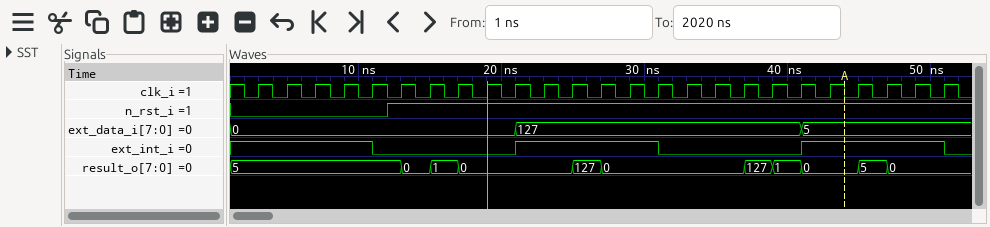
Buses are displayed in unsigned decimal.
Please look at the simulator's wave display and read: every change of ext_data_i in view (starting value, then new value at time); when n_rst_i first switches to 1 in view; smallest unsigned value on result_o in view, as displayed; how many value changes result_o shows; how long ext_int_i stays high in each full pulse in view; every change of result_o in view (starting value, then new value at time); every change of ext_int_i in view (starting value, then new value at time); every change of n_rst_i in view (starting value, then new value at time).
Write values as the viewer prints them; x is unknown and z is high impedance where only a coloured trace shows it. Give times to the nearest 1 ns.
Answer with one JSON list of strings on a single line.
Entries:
["0, 127 at 21 ns, 5 at 41 ns", "12 ns", "0", "10", "10 ns, 10 ns", "5, 0 at 13 ns, 1 at 15 ns, 0 at 17 ns, 127 at 25 ns, 0 at 27 ns, 127 at 37 ns, 1 at 39 ns, 0 at 41 ns, 5 at 45 ns, 0 at 47 ns", "1, 0 at 11 ns, 1 at 21 ns, 0 at 31 ns, 1 at 41 ns, 0 at 51 ns", "0, 1 at 12 ns"]
